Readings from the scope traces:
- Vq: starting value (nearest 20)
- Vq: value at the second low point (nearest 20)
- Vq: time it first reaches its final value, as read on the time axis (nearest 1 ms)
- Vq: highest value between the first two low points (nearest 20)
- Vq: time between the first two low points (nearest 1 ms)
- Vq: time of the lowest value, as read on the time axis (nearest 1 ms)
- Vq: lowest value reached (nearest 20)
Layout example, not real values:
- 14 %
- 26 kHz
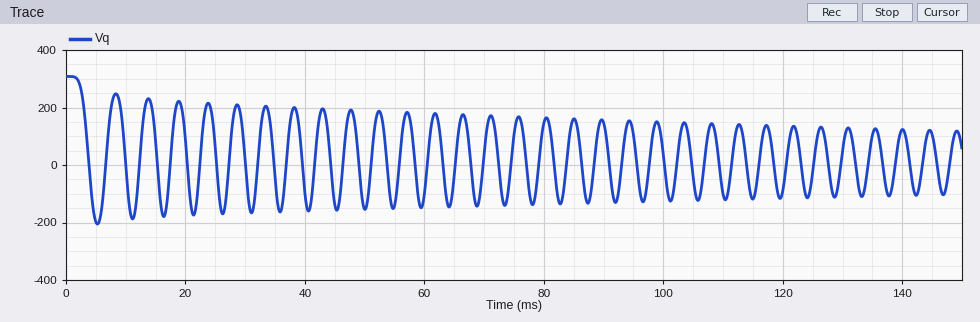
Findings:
- 300
- -180
- 4 ms
- 240
- 6 ms
- 5 ms
- -200
